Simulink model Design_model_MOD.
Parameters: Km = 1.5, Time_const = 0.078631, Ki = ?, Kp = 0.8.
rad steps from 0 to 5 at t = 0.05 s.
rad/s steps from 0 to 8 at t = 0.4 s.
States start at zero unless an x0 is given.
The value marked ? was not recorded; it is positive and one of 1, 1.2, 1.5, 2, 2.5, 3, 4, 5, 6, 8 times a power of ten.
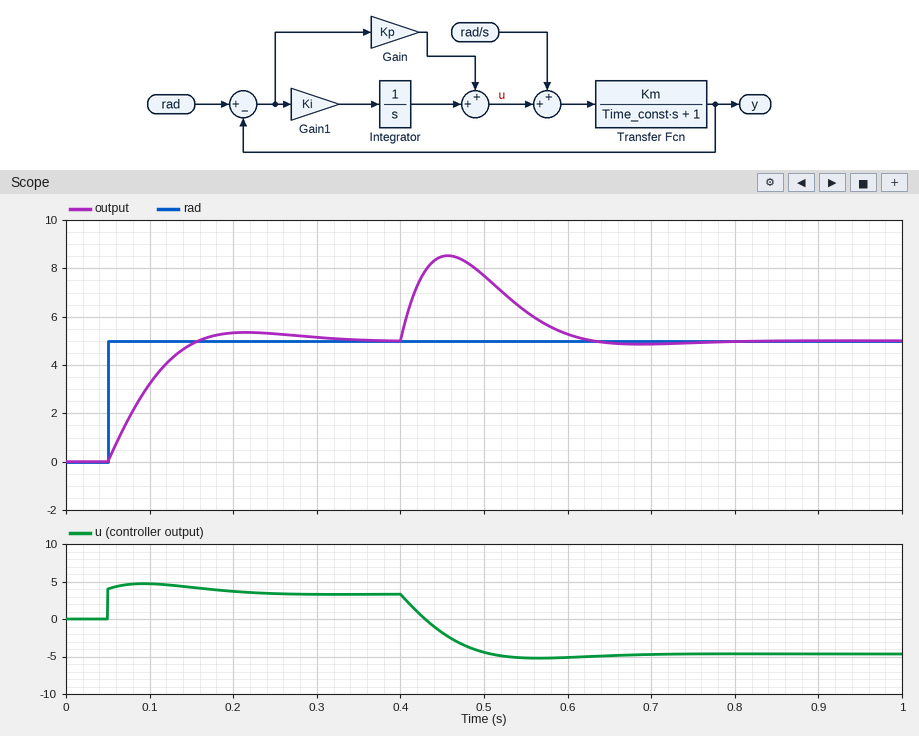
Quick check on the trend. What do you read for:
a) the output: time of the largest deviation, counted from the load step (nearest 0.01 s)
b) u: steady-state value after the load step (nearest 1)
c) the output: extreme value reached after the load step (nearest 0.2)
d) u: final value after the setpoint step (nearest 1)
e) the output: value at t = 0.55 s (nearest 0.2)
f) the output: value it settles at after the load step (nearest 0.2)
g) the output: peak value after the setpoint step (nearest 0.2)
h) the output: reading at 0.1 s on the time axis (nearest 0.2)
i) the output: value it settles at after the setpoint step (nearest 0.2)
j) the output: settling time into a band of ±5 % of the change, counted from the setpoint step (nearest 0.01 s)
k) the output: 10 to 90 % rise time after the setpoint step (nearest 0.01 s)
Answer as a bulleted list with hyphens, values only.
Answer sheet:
- 0.06 s
- -5
- 8.6
- 3
- 6.2
- 5.0
- 5.4
- 3.2
- 5.0
- 0.21 s
- 0.08 s
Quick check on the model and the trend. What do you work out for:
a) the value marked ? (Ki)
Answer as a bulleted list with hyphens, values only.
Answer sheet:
- 20
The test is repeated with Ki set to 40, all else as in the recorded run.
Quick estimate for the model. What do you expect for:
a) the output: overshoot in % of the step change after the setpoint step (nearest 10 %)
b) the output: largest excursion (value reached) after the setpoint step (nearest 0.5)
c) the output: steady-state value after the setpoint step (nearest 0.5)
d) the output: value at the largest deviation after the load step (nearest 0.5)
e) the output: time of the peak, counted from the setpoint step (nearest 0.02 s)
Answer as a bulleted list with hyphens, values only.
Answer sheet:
- 20 %
- 6.0
- 5.0
- 8.0
- 0.10 s
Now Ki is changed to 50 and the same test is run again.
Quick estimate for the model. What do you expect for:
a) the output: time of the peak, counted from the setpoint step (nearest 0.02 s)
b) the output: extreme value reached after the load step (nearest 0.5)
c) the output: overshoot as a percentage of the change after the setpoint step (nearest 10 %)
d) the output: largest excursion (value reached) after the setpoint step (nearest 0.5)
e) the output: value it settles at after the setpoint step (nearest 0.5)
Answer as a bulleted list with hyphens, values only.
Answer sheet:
- 0.10 s
- 8.0
- 20 %
- 6.0
- 5.0
